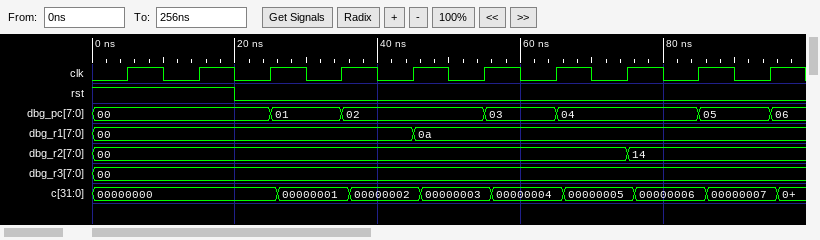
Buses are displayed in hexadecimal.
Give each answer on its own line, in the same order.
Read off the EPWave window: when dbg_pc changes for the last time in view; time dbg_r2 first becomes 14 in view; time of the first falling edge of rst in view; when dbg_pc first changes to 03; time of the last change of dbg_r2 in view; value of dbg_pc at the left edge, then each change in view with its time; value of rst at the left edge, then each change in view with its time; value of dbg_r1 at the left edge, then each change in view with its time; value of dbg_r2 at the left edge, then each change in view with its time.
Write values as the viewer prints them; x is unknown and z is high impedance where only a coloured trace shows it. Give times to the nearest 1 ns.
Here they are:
95 ns
75 ns
20 ns
55 ns
75 ns
00, 01 at 25 ns, 02 at 35 ns, 03 at 55 ns, 04 at 65 ns, 05 at 85 ns, 06 at 95 ns
1, 0 at 20 ns
00, 0a at 45 ns
00, 14 at 75 ns
